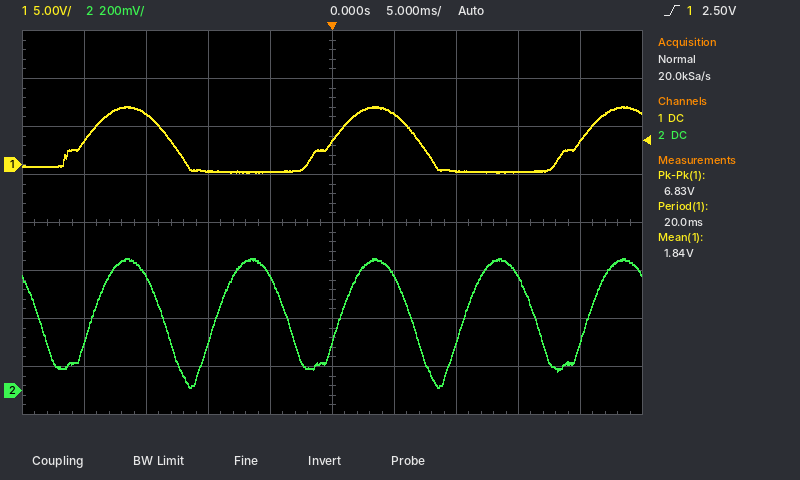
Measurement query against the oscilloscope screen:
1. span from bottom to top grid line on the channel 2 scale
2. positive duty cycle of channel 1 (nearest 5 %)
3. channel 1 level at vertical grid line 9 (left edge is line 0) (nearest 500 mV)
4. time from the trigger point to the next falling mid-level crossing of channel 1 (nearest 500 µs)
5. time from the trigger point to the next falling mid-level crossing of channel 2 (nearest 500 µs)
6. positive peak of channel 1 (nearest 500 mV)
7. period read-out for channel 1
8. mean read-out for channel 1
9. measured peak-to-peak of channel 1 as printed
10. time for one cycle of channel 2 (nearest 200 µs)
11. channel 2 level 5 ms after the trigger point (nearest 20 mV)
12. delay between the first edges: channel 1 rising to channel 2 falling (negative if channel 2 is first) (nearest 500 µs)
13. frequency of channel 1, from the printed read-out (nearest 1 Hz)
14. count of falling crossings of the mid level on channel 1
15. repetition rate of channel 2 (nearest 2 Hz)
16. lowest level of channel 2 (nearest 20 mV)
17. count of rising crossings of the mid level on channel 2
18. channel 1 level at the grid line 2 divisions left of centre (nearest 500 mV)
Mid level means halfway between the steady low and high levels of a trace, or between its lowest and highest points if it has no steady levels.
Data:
1.6 V
35 %
2.5 V
7.0 ms
6.5 ms
6.0 V
20.0 ms
1.84 V
6.83 V
10.0 ms
480 mV
-3.5 ms
50 Hz
2
100 Hz
20 mV
5
-500 mV
